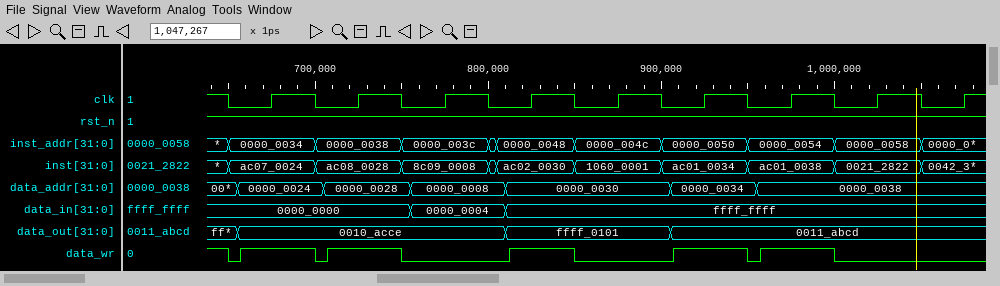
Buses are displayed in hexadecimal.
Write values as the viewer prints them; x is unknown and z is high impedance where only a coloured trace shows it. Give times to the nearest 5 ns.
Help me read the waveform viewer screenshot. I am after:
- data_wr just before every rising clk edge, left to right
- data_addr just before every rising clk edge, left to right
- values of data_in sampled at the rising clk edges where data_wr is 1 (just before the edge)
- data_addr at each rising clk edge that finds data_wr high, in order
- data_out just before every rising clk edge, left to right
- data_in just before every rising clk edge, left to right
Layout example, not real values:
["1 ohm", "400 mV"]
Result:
["1 1 0 1 0 1 1 0 0", "0000_0024, 0000_0028, 0000_0008, 0000_0030, 0000_0030, 0000_0034, 0000_0038, 0000_0038, 0000_0038", "0000_0000, 0000_0000, ffff_ffff, ffff_ffff, ffff_ffff", "0000_0024, 0000_0028, 0000_0030, 0000_0034, 0000_0038", "0010_acce, 0010_acce, 0010_acce, ffff_0101, ffff_0101, 0011_abcd, 0011_abcd, 0011_abcd, 0011_abcd", "0000_0000, 0000_0000, 0000_0004, ffff_ffff, ffff_ffff, ffff_ffff, ffff_ffff, ffff_ffff, ffff_ffff"]
